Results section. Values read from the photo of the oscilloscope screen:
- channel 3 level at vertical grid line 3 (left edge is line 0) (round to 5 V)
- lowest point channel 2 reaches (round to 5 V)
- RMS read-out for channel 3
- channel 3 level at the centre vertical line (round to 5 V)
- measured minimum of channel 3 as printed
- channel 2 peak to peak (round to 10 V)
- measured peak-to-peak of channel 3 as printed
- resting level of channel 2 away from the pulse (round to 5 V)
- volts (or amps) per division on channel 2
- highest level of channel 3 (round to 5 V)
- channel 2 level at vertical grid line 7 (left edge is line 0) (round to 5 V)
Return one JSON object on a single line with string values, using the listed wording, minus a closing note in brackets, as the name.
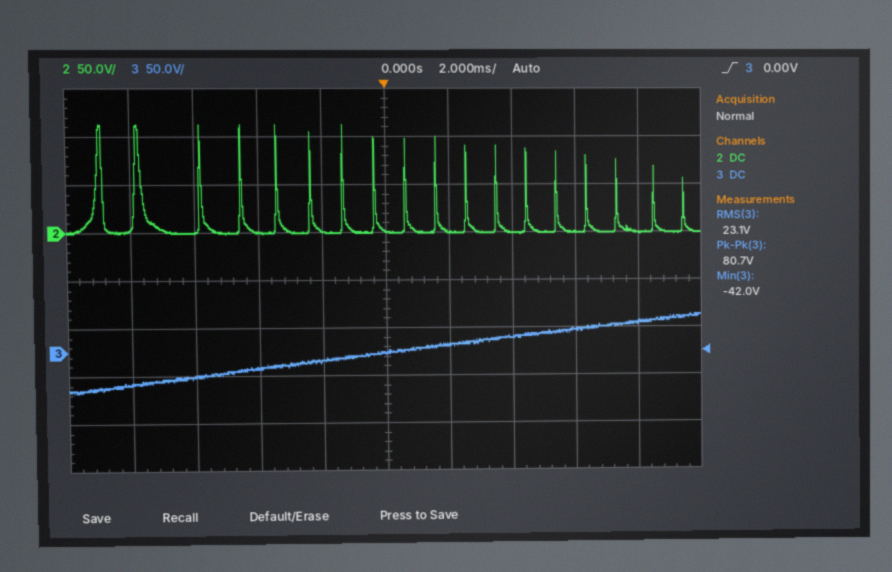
{"channel 3 level at vertical grid line 3 (left edge is line 0)": "-15 V", "lowest point channel 2 reaches": "0 V", "RMS read-out for channel 3": "23.1 V", "channel 3 level at the centre vertical line": "0 V", "measured minimum of channel 3 as printed": "-42.0 V", "channel 2 peak to peak": "110 V", "measured peak-to-peak of channel 3 as printed": "80.7 V", "resting level of channel 2 away from the pulse": "0 V", "volts (or amps) per division on channel 2": "50 V", "highest level of channel 3": "40 V", "channel 2 level at vertical grid line 7 (left edge is line 0)": "0 V"}
